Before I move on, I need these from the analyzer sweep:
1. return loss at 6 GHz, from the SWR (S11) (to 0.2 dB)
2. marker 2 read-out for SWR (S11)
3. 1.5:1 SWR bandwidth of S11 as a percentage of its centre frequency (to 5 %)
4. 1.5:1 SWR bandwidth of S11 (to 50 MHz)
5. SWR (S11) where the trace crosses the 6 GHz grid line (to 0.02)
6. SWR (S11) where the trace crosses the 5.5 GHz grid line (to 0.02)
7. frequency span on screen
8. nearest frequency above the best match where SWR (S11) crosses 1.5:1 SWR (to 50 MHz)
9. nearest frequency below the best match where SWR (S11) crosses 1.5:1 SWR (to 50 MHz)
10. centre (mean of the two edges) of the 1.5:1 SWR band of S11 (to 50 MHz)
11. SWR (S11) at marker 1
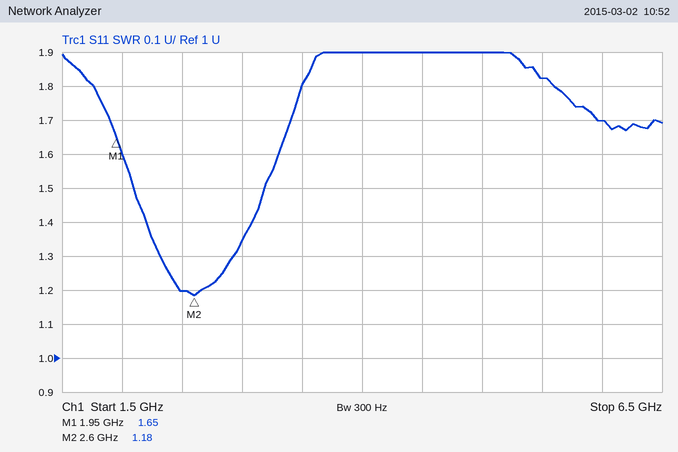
11.8 dB
1.18
40 %
1.10 GHz
1.70
1.82
5 GHz
3.20 GHz
2.10 GHz
2.65 GHz
1.65
